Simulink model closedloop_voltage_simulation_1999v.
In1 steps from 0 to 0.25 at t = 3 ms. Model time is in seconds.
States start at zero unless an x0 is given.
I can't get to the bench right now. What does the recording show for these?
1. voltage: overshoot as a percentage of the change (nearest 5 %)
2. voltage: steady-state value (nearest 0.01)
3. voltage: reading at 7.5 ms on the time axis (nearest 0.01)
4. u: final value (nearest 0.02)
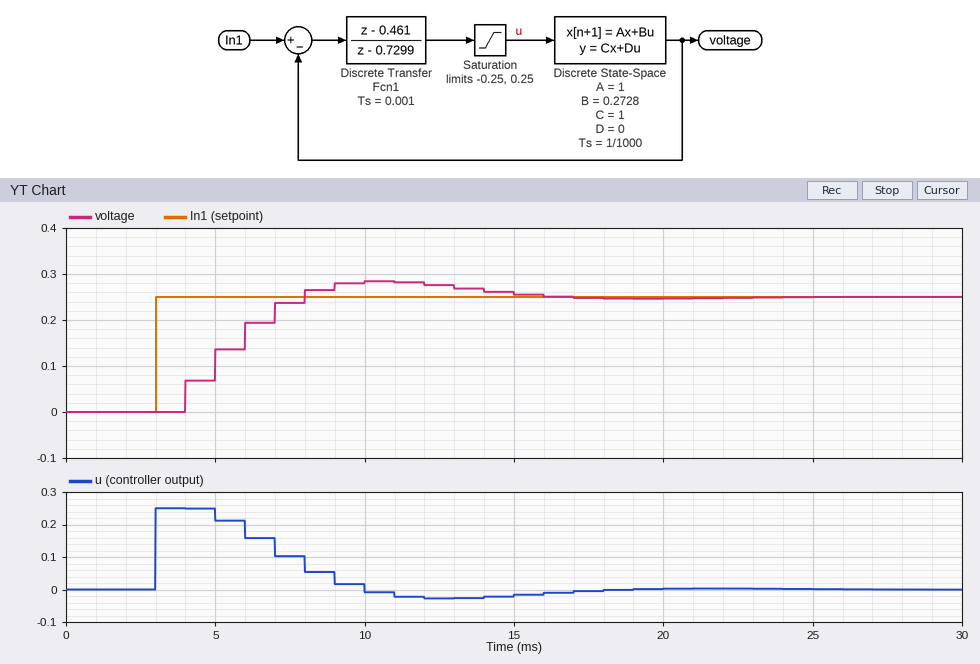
15 %
0.25
0.24
0.00
